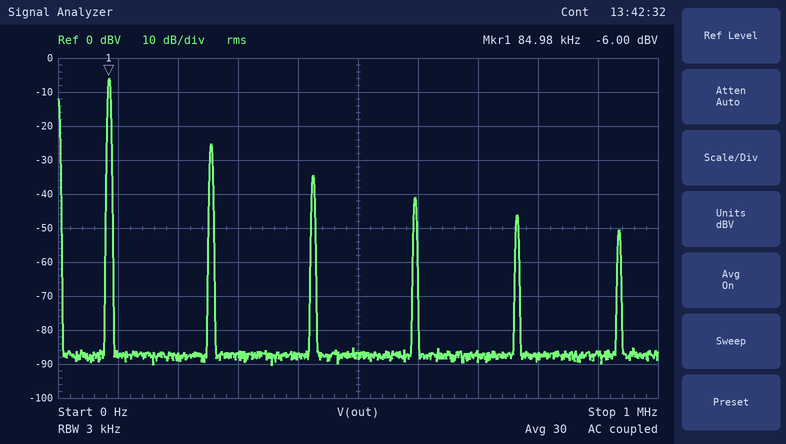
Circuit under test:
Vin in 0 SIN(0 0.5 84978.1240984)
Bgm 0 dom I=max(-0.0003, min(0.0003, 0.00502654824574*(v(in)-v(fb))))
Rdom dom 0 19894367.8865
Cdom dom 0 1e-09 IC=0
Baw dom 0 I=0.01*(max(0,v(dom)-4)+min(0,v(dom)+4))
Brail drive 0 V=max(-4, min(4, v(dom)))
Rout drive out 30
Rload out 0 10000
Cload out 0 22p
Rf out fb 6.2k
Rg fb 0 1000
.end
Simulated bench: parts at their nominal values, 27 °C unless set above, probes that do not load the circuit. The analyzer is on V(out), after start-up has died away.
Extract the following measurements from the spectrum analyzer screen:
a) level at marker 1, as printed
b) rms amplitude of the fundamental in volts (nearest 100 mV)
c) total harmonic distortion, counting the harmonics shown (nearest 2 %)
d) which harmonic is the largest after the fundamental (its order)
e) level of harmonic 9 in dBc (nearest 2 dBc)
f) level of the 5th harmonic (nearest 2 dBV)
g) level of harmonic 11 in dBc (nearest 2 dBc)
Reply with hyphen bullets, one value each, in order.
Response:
- -6.00 dBV
- 500 mV
- 12 %
- 3
- -40 dBc
- -34 dBV
- -44 dBc
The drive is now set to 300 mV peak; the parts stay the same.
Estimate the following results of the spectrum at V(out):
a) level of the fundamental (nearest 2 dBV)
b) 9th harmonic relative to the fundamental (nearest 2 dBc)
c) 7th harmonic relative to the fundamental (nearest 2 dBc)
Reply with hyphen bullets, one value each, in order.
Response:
- -6 dBV
- -44 dBc
- -38 dBc
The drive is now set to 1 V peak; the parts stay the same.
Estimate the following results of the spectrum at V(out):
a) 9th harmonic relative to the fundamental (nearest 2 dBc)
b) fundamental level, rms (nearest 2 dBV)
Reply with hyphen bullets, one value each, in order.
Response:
- -38 dBc
- -6 dBV
